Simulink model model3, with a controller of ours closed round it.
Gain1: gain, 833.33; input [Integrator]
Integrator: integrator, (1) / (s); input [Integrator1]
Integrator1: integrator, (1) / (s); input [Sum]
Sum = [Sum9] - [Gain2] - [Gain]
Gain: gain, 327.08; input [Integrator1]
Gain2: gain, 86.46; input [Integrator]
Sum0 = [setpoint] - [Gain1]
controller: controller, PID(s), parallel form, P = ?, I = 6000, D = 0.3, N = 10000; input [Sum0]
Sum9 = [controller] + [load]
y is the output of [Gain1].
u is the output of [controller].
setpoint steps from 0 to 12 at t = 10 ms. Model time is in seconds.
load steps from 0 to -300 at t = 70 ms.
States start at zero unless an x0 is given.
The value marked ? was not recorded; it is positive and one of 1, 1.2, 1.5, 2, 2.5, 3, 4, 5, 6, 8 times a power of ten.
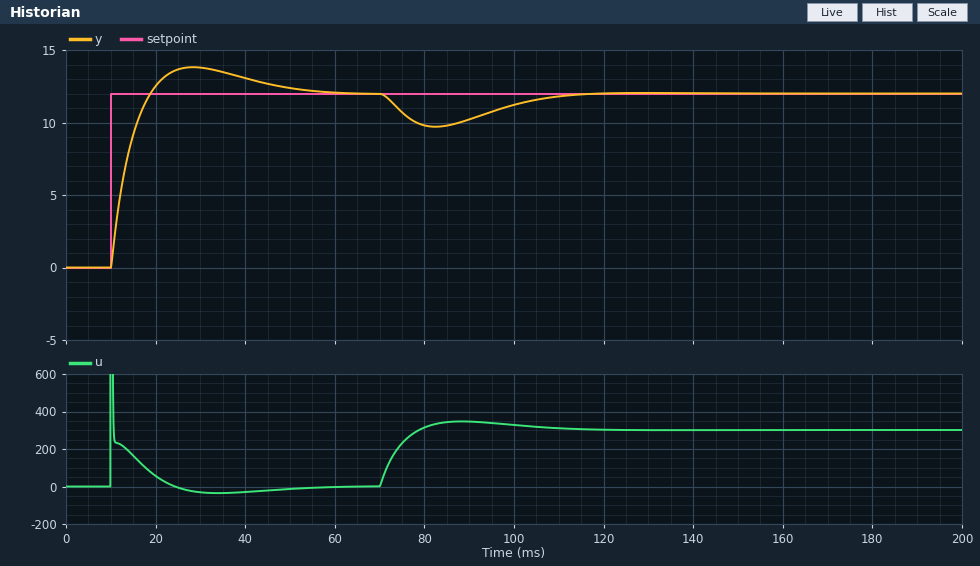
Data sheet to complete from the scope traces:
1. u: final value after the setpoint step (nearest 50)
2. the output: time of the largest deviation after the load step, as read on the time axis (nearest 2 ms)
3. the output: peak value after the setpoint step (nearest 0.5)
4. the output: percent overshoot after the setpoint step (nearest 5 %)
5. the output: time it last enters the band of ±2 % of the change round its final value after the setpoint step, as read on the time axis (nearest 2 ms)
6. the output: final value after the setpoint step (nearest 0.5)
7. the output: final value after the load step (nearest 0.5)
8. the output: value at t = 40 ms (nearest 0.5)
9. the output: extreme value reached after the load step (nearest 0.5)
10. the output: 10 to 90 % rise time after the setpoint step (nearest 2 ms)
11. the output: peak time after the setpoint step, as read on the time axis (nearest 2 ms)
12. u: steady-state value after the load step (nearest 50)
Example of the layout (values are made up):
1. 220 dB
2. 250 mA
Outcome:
1. 0
2. 82 ms
3. 14.0
4. 15 %
5. 54 ms
6. 12.0
7. 12.0
8. 13.0
9. 9.5
10. 6 ms
11. 28 ms
12. 300
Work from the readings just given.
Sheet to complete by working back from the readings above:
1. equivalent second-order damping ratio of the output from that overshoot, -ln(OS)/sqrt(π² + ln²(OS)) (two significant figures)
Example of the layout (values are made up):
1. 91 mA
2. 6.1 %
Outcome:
1. 0.52
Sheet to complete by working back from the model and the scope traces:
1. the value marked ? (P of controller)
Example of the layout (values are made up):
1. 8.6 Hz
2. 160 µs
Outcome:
1. 100
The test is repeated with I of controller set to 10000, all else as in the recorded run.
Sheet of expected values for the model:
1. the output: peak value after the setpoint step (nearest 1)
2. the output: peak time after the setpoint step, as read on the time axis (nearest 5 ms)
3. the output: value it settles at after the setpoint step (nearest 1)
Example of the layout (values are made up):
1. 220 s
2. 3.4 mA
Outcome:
1. 15
2. 25 ms
3. 12
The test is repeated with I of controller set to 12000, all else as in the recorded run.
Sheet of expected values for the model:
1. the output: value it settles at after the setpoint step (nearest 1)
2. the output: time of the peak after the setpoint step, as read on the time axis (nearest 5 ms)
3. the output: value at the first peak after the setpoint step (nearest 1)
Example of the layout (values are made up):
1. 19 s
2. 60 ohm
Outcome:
1. 12
2. 25 ms
3. 15
